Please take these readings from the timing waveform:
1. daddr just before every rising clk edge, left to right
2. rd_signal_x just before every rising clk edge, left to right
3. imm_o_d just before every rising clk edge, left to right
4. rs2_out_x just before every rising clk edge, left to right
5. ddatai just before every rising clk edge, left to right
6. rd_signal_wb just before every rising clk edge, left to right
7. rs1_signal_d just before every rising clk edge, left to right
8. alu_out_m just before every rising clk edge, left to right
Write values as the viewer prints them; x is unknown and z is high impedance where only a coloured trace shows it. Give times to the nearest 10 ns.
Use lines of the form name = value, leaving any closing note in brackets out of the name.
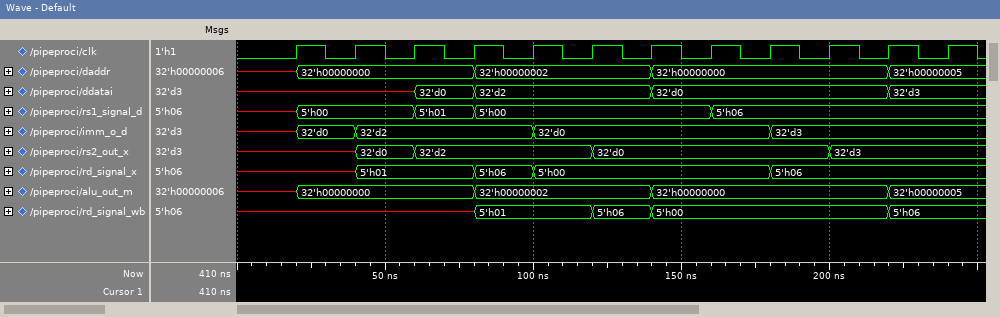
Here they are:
daddr just before every rising clk edge, left to right = x, 32'h00000000, 32'h00000000, 32'h00000000, 32'h00000002, 32'h00000002, 32'h00000002, 32'h00000000, 32'h00000000, 32'h00000000, 32'h00000000, 32'h00000005
rd_signal_x just before every rising clk edge, left to right = x, x, 5'h01, 5'h01, 5'h06, 5'h00, 5'h00, 5'h00, 5'h00, 5'h06, 5'h06, 5'h06
imm_o_d just before every rising clk edge, left to right = x, 32'd0, 32'd2, 32'd2, 32'd2, 32'd0, 32'd0, 32'd0, 32'd0, 32'd3, 32'd3, 32'd3
rs2_out_x just before every rising clk edge, left to right = x, x, 32'd0, 32'd2, 32'd2, 32'd2, 32'd0, 32'd0, 32'd0, 32'd0, 32'd3, 32'd3
ddatai just before every rising clk edge, left to right = x, x, x, 32'd0, 32'd2, 32'd2, 32'd2, 32'd0, 32'd0, 32'd0, 32'd0, 32'd3
rd_signal_wb just before every rising clk edge, left to right = x, x, x, x, 5'h01, 5'h01, 5'h06, 5'h00, 5'h00, 5'h00, 5'h00, 5'h06
rs1_signal_d just before every rising clk edge, left to right = x, 5'h00, 5'h00, 5'h01, 5'h00, 5'h00, 5'h00, 5'h00, 5'h06, 5'h06, 5'h06, 5'h06
alu_out_m just before every rising clk edge, left to right = x, 32'h00000000, 32'h00000000, 32'h00000000, 32'h00000002, 32'h00000002, 32'h00000002, 32'h00000000, 32'h00000000, 32'h00000000, 32'h00000000, 32'h00000005
